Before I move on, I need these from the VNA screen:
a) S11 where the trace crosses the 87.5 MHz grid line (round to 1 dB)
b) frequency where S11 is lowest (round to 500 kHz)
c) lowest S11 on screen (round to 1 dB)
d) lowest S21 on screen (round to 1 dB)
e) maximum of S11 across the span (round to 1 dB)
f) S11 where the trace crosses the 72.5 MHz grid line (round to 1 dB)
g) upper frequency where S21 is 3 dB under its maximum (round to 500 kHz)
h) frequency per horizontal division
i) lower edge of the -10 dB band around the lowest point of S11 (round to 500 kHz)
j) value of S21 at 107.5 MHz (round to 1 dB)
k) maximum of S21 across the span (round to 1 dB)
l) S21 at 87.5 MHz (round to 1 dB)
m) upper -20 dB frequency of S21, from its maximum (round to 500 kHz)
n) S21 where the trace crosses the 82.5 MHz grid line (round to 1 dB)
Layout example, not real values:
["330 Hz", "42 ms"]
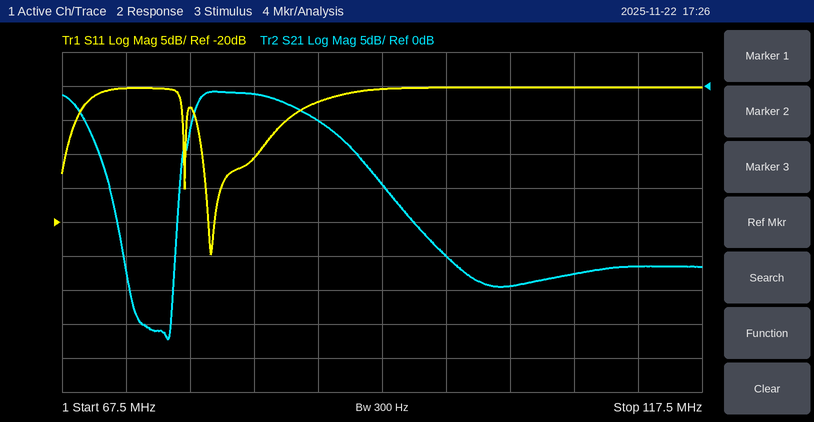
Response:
["-2 dB", "79.0 MHz", "-25 dB", "-37 dB", "0 dB", "0 dB", "86.5 MHz", "5 MHz", "78.5 MHz", "-28 dB", "-1 dB", "-5 dB", "95.5 MHz", "-1 dB"]
